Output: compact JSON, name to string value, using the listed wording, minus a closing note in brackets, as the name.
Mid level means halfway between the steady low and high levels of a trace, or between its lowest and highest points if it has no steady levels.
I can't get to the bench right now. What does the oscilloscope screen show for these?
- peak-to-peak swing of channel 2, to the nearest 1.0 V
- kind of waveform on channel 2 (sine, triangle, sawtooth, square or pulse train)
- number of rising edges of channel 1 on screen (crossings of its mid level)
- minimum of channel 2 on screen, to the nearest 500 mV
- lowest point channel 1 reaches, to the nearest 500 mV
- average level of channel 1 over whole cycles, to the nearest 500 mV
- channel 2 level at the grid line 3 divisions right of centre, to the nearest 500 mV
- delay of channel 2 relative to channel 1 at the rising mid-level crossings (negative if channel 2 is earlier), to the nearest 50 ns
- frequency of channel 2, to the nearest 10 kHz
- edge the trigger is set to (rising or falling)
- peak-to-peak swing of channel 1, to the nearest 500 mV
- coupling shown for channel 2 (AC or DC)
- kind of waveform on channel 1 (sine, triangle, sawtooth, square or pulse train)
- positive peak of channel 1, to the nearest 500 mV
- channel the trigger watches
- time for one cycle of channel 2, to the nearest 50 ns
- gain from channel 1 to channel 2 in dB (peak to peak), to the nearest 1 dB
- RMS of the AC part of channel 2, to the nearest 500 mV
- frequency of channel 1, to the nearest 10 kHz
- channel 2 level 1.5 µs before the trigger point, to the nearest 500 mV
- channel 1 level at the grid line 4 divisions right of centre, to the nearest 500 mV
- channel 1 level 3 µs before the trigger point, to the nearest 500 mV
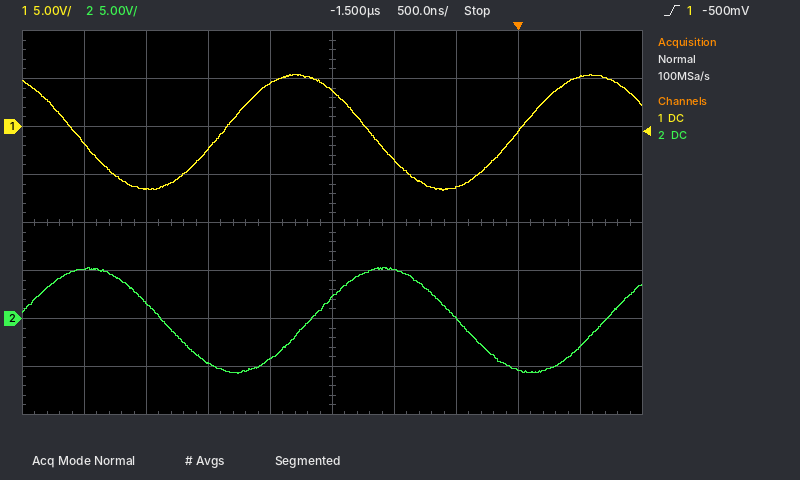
{"peak-to-peak swing of channel 2, to the nearest 1.0 V": "11.0 V", "kind of waveform on channel 2": "sine", "number of rising edges of channel 1 on screen": "2", "minimum of channel 2 on screen, to the nearest 500 mV": "-5.5 V", "lowest point channel 1 reaches, to the nearest 500 mV": "-6.5 V", "average level of channel 1 over whole cycles, to the nearest 500 mV": "-500 mV", "channel 2 level at the grid line 3 divisions right of centre, to the nearest 500 mV": "-5.5 V", "delay of channel 2 relative to channel 1 at the rising mid-level crossings (negative if channel 2 is earlier), to the nearest 50 ns": "+700 ns", "frequency of channel 2, to the nearest 10 kHz": "420 kHz", "edge the trigger is set to": "rising", "peak-to-peak swing of channel 1, to the nearest 500 mV": "12.0 V", "coupling shown for channel 2": "DC", "kind of waveform on channel 1": "sine", "positive peak of channel 1, to the nearest 500 mV": "5.5 V", "channel the trigger watches": "channel 1", "time for one cycle of channel 2, to the nearest 50 ns": "2.40 µs", "gain from channel 1 to channel 2 in dB (peak to peak), to the nearest 1 dB": "-1 dB", "RMS of the AC part of channel 2, to the nearest 500 mV": "4.0 V", "frequency of channel 1, to the nearest 10 kHz": "420 kHz", "channel 2 level 1.5 µs before the trigger point, to the nearest 500 mV": "2.0 V", "channel 1 level at the grid line 4 divisions right of centre, to the nearest 500 mV": "5.0 V", "channel 1 level 3 µs before the trigger point, to the nearest 500 mV": "-6.5 V"}
